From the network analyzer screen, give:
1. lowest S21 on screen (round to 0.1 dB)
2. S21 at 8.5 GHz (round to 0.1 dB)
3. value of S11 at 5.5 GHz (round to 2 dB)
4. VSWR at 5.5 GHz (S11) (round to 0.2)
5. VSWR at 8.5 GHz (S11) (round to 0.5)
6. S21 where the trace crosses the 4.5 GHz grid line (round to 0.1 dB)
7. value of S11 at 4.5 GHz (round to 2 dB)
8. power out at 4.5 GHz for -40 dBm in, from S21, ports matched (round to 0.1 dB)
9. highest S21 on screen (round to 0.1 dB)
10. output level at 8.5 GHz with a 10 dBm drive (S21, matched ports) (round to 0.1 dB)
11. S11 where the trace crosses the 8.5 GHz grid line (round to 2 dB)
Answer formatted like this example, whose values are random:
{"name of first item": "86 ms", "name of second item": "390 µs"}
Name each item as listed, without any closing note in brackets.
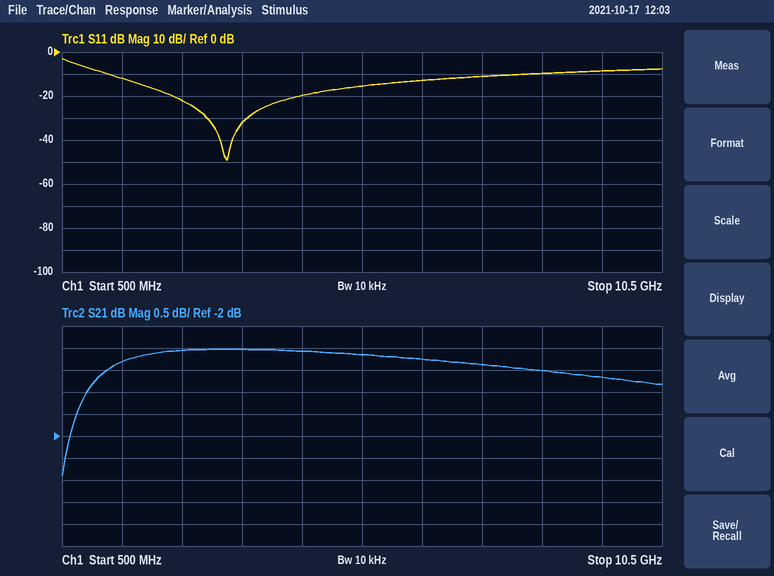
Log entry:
{"lowest S21 on screen": "-2.9 dB", "S21 at 8.5 GHz": "-0.5 dB", "value of S11 at 5.5 GHz": "-16 dB", "VSWR at 5.5 GHz (S11)": "1.4", "VSWR at 8.5 GHz (S11)": "2.0", "S21 where the trace crosses the 4.5 GHz grid line": "-0.1 dB", "value of S11 at 4.5 GHz": "-20 dB", "power out at 4.5 GHz for -40 dBm in, from S21, ports matched": "-40.1 dBm", "highest S21 on screen": "0.0 dB", "output level at 8.5 GHz with a 10 dBm drive (S21, matched ports)": "9.5 dBm", "S11 where the trace crosses the 8.5 GHz grid line": "-10 dB"}
